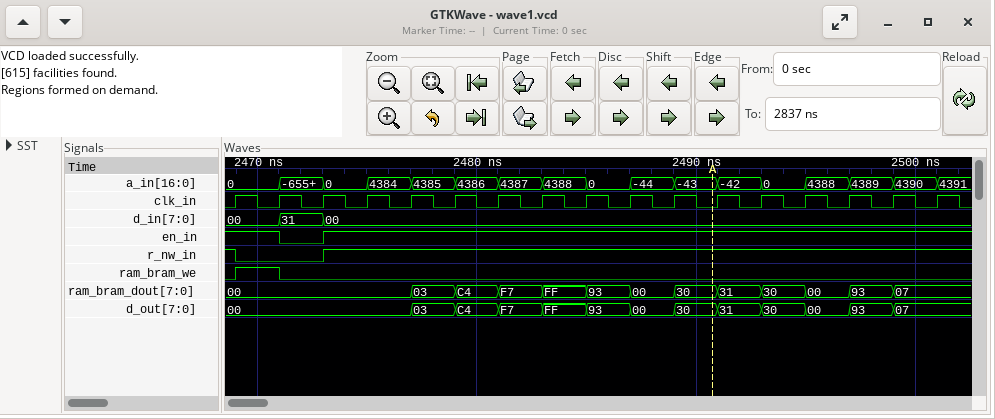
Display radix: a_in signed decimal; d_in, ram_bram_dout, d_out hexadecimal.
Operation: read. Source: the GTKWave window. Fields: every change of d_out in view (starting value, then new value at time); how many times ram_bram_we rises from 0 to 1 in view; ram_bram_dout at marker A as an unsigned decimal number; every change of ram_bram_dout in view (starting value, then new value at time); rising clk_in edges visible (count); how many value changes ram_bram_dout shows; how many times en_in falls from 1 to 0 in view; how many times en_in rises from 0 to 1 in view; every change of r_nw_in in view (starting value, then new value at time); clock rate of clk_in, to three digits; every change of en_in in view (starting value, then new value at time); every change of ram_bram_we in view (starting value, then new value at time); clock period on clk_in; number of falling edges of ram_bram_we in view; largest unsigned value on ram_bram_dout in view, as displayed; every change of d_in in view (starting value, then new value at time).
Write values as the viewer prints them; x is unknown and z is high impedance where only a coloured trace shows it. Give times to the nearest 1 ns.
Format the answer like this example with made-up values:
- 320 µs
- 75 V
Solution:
- 00, 03 at 2477 ns, C4 at 2479 ns, F7 at 2481 ns, FF at 2483 ns, 93 at 2485 ns, 00 at 2487 ns, 30 at 2489 ns, 31 at 2491 ns, 30 at 2493 ns, 00 at 2495 ns, 93 at 2497 ns, 07 at 2499 ns
- 1
- 48
- 00, 03 at 2477 ns, C4 at 2479 ns, F7 at 2481 ns, FF at 2483 ns, 93 at 2485 ns, 00 at 2487 ns, 30 at 2489 ns, 31 at 2491 ns, 30 at 2493 ns, 00 at 2495 ns, 93 at 2497 ns, 07 at 2499 ns
- 17
- 12
- 1
- 1
- 1, 0 at 2469 ns, 1 at 2473 ns
- 500 MHz
- 1, 0 at 2471 ns, 1 at 2473 ns
- 0, 1 at 2469 ns, 0 at 2471 ns
- 2 ns
- 1
- FF
- 00, 31 at 2471 ns, 00 at 2473 ns
